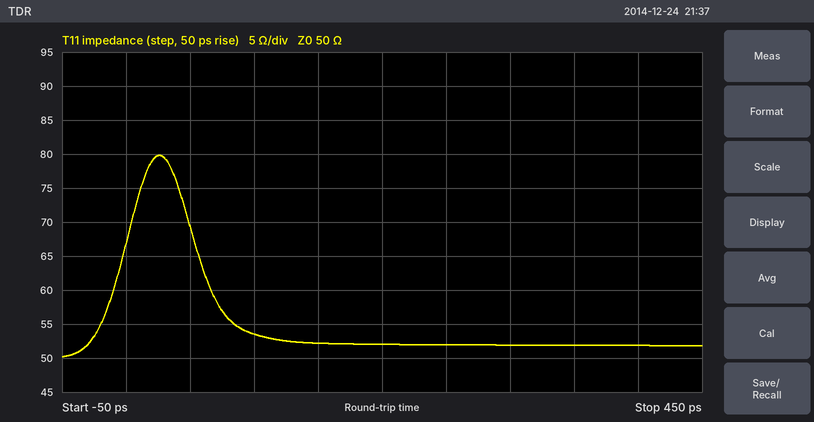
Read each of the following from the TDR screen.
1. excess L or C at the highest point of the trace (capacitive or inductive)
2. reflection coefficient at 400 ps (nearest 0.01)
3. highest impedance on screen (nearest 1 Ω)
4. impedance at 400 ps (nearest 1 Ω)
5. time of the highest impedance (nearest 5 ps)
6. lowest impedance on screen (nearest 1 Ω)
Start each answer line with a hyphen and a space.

- inductive
- +0.02
- 80 Ω
- 52 Ω
- 25 ps
- 50 Ω
